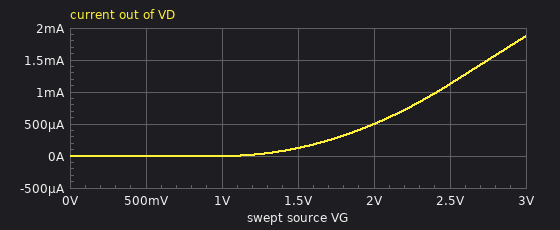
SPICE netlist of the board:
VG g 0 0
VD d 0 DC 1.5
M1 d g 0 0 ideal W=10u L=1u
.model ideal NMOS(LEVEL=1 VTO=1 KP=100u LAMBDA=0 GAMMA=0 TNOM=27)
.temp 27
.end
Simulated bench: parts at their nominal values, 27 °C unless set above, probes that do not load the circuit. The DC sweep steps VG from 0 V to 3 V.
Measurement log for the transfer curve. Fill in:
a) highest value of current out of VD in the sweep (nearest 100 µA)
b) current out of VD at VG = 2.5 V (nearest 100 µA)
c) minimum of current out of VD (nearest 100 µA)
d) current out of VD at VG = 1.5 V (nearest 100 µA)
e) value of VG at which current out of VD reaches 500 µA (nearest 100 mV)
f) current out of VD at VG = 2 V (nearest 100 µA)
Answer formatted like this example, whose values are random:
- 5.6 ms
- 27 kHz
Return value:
- 1.9 mA
- 1.1 mA
- 0 A
- 100 µA
- 2.0 V
- 500 µA
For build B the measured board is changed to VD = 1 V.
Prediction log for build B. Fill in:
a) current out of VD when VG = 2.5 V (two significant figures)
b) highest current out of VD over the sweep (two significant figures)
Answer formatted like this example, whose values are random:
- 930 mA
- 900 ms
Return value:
- 1.0 mA
- 1.5 mA
